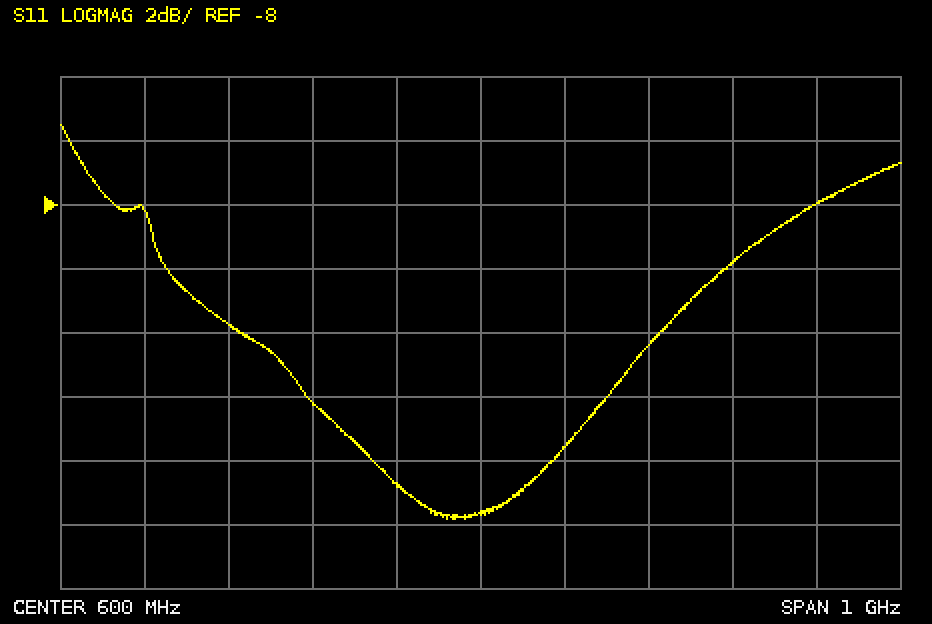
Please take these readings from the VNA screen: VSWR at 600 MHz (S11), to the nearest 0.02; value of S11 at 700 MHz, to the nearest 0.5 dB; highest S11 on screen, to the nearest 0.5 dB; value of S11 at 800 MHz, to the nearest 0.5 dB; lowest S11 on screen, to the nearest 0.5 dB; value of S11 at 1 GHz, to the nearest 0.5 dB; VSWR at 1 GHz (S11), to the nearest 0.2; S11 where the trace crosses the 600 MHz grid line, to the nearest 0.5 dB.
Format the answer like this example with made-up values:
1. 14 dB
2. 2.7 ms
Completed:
1. 1.30
2. -15.5 dB
3. -5.5 dB
4. -12.5 dB
5. -18.0 dB
6. -8.0 dB
7. 2.4
8. -17.5 dB
